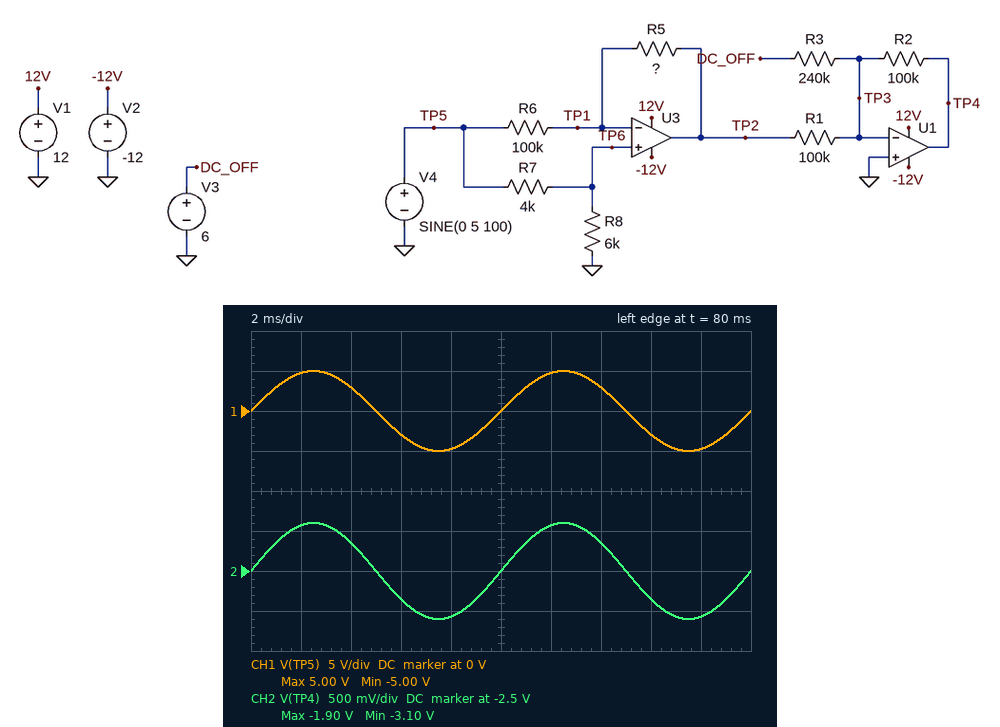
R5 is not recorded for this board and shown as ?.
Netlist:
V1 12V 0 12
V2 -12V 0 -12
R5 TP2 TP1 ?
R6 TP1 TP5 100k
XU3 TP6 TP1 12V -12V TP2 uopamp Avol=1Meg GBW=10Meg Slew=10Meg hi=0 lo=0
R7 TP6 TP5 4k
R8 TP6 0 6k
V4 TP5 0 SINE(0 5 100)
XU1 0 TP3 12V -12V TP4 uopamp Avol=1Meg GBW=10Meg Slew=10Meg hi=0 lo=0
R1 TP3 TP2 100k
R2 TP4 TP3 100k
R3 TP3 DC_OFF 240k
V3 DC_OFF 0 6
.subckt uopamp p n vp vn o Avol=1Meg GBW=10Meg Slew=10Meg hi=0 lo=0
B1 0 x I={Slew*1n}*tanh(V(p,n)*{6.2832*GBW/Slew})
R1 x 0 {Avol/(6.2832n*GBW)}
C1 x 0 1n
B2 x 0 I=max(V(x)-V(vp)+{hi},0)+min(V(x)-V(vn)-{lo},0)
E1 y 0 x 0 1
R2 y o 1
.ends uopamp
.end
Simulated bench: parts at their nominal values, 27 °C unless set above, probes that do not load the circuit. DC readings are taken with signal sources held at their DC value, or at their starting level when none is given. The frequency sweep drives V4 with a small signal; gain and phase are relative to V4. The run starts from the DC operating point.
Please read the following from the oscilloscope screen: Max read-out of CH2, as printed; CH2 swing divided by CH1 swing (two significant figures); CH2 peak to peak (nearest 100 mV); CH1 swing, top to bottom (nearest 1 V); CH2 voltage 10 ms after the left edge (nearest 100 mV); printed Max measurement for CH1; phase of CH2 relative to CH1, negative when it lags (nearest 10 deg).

-1.90 V
0.12
1.2 V
10 V
-2.5 V
5.00 V
0 deg
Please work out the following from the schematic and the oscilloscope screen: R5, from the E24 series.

180 kΩ
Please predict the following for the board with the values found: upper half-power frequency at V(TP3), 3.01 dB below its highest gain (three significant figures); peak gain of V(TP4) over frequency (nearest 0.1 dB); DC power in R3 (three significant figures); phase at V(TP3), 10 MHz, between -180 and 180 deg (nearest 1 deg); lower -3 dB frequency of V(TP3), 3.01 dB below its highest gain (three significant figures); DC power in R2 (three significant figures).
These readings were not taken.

9.30 MHz
-18.4 dB
150 µW
132 deg
1.59 MHz
62.5 µW
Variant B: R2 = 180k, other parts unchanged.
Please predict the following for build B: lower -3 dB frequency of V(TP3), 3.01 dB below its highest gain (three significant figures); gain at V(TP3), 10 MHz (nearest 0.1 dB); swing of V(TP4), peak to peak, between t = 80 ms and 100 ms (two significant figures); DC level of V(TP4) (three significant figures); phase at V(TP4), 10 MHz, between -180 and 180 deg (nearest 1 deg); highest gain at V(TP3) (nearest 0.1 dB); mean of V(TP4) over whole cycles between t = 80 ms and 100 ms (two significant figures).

1.31 MHz
-34.1 dB
2.2 V
-4.50 V
-145 deg
-29.4 dB
-4.5 V
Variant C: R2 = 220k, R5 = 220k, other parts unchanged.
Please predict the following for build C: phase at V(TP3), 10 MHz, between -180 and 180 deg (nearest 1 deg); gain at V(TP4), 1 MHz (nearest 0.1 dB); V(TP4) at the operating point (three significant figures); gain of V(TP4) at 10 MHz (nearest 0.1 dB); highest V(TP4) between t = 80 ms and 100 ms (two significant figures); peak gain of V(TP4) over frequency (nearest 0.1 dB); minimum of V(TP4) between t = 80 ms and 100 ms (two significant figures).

121 deg
-5.3 dB
-5.50 V
-27.3 dB
-2.4 V
-4.2 dB
-8.6 V
